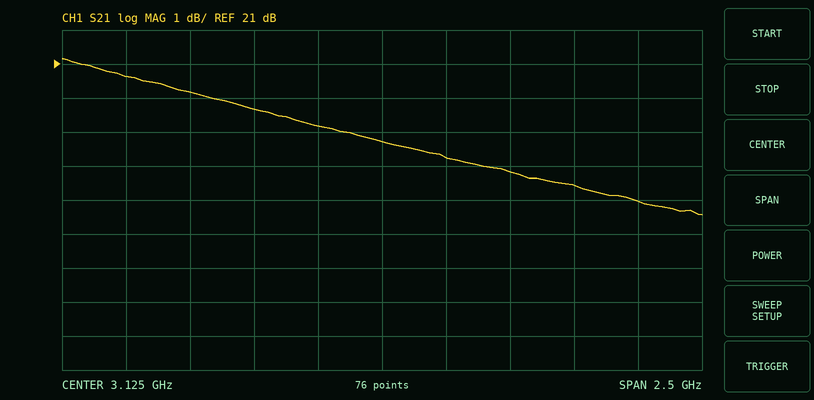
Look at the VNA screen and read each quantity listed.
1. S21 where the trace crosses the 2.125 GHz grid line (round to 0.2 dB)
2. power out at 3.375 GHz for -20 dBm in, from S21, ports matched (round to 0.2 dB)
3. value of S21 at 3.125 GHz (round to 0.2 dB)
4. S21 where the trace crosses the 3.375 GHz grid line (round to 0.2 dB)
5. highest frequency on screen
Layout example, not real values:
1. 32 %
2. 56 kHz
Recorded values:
1. 20.6 dB
2. -1.8 dBm
3. 18.8 dB
4. 18.2 dB
5. 4.375 GHz
